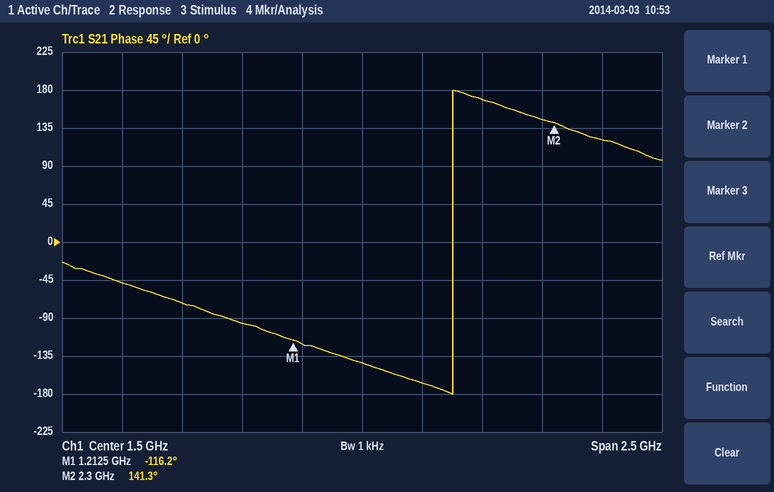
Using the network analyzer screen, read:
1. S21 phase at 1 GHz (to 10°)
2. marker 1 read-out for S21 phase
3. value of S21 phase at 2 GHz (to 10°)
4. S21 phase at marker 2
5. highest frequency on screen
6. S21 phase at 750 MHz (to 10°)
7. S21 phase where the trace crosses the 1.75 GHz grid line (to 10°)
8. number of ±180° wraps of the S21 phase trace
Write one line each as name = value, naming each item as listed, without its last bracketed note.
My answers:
S21 phase at 1 GHz = -100°
marker 1 read-out for S21 phase = -116.2°
value of S21 phase at 2 GHz = 170°
S21 phase at marker 2 = 141.3°
highest frequency on screen = 2.75 GHz
S21 phase at 750 MHz = -70°
S21 phase where the trace crosses the 1.75 GHz grid line = -170°
number of ±180° wraps of the S21 phase trace = 1
